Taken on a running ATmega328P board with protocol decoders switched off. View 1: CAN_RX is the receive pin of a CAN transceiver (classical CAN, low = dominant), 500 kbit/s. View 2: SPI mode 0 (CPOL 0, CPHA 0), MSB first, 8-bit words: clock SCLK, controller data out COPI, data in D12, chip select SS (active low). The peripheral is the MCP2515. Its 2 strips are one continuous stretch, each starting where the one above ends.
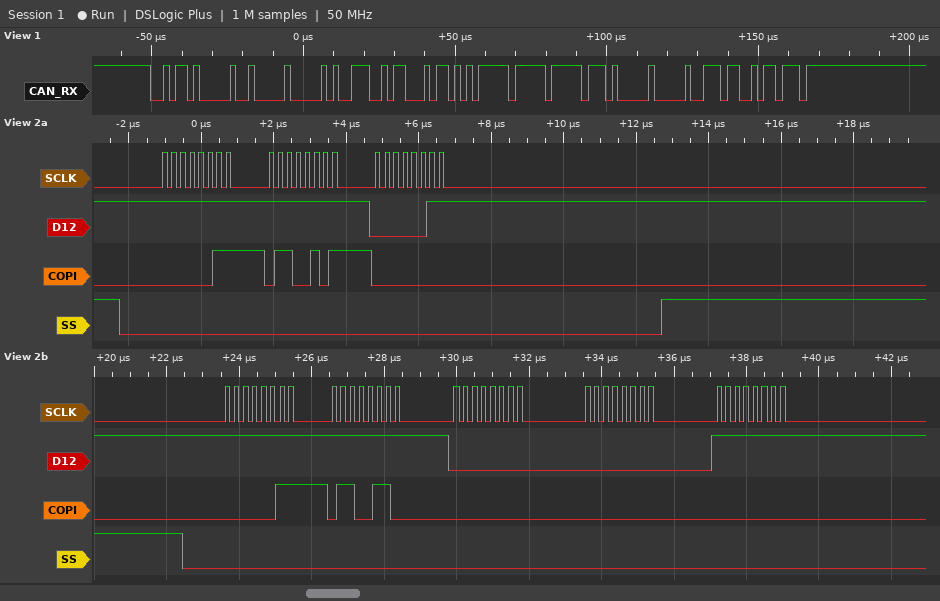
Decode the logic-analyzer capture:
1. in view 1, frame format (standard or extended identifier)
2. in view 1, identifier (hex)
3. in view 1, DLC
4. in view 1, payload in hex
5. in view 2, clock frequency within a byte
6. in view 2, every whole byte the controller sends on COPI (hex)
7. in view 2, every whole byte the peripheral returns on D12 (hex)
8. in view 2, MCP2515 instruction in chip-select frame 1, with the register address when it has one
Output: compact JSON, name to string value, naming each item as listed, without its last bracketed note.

{"in view 1, frame format": "standard", "in view 1, identifier": "0x2D0", "in view 1, DLC": "8", "in view 1, payload in hex": "00 9C B1 6A FF FF D0 00", "in view 2, clock frequency within a byte": "4 MHz", "in view 2, every whole byte the controller sends on COPI": "03 65 00 03 66 00 00 00", "in view 2, every whole byte the peripheral returns on D12": "FF FF 03 FF FF 00 00 FF", "in view 2, MCP2515 instruction in chip-select frame 1, with the register address when it has one": "READ 0x65"}
